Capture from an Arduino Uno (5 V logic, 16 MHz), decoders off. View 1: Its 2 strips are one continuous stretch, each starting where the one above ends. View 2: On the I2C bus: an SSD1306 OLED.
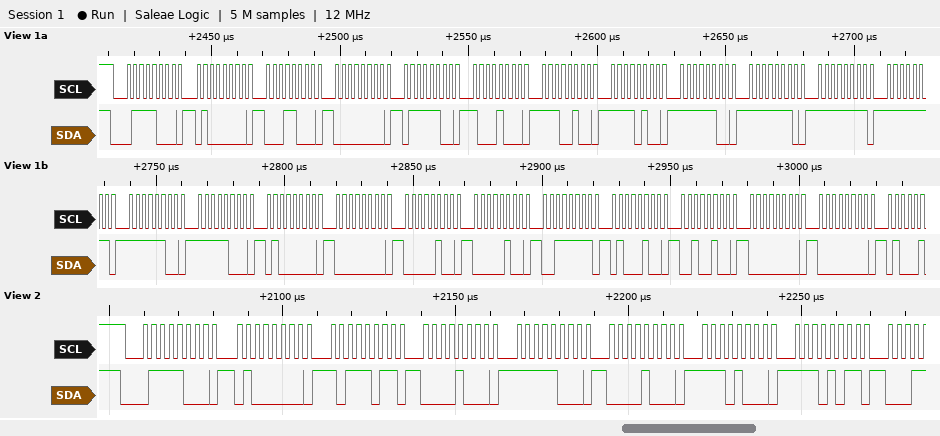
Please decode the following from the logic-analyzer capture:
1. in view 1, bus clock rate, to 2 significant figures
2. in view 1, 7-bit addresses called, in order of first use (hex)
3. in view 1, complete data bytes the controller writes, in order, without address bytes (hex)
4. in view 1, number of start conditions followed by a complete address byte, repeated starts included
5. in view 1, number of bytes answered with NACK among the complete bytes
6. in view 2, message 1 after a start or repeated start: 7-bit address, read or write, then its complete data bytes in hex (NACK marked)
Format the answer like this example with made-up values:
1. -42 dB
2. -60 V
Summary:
1. 400 kHz
2. 0x3C
3. 40 18 00 7C 88 E4 F4 FC FE FF FF FC F8 40 00 04 04 3F 44 24 00 00
4. 1
5. 0
6. 0x3C write: 40 BB 08 F8 08 E8 EB
